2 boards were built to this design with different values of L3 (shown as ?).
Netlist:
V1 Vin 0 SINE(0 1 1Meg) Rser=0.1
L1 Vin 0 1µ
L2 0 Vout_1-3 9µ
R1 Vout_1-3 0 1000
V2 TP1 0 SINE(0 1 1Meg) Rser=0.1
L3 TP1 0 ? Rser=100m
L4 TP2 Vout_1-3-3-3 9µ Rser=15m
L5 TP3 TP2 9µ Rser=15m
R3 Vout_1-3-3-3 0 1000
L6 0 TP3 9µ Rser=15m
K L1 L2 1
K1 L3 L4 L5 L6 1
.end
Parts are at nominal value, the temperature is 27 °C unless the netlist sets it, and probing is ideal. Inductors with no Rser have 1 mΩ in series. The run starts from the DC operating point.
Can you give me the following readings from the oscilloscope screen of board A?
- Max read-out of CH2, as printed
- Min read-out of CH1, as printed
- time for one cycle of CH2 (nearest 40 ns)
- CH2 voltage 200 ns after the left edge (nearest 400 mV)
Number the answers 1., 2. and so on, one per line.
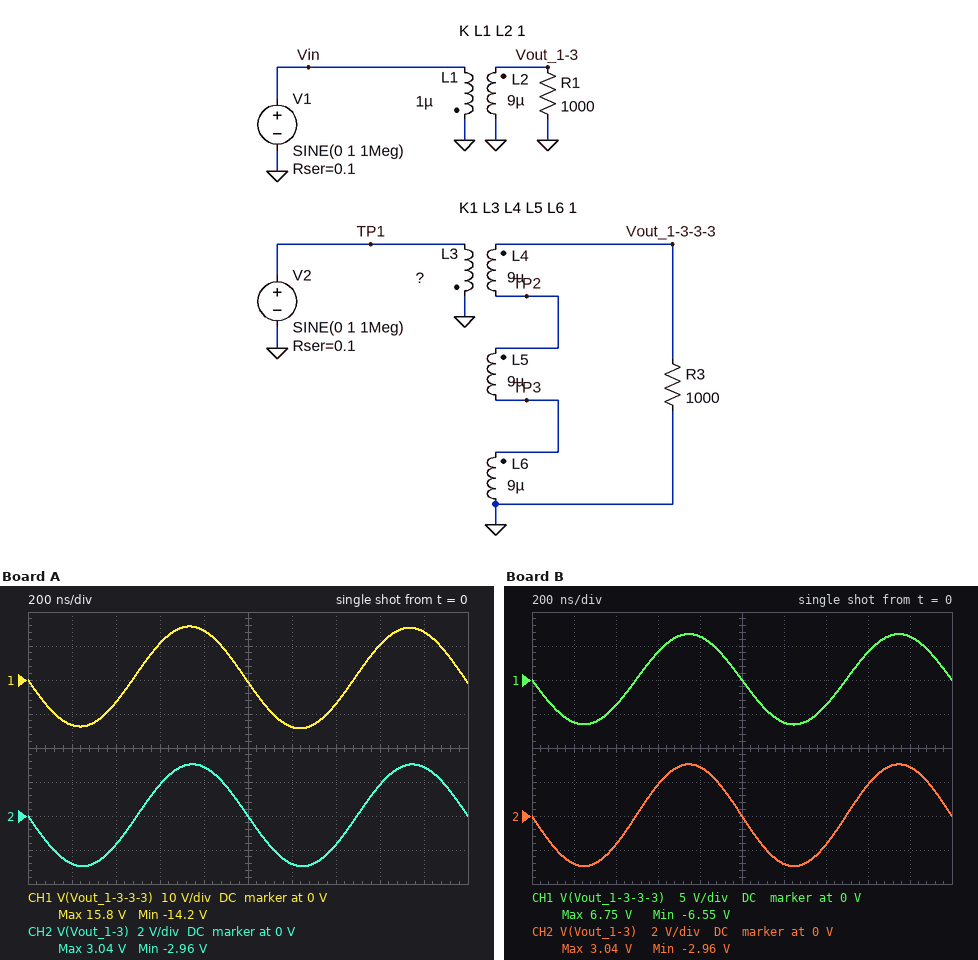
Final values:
1. 3.04 V
2. -14.2 V
3. 1.00 µs
4. -2.8 V
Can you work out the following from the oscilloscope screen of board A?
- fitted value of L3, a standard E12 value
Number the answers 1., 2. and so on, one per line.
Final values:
1. 330 nH
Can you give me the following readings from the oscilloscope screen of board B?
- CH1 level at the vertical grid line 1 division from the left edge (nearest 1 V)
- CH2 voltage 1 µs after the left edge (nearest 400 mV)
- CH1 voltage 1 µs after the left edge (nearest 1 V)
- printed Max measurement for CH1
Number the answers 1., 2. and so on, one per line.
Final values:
1. -6 V
2. 0 V
3. 0 V
4. 6.75 V
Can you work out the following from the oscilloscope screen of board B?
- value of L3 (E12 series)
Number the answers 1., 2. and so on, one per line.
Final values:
1. 1.8 µH
